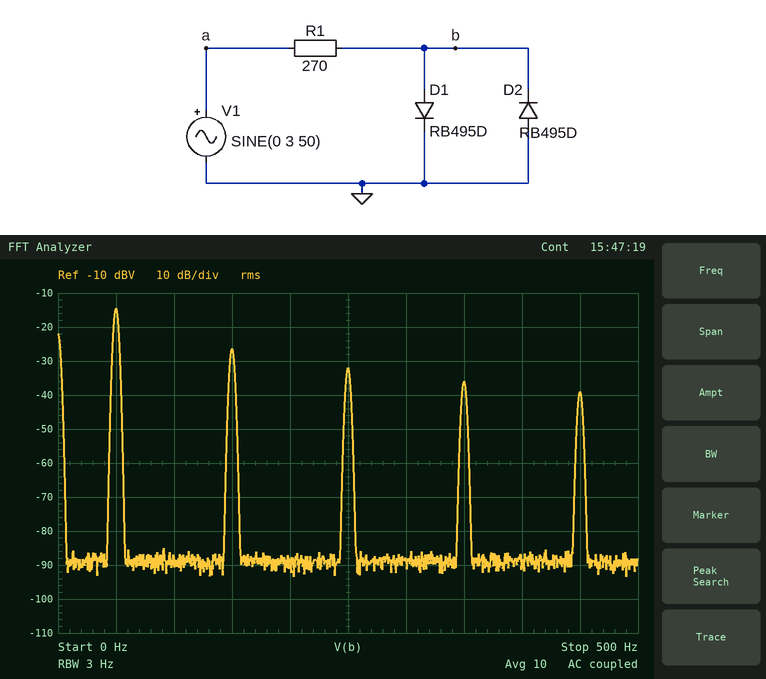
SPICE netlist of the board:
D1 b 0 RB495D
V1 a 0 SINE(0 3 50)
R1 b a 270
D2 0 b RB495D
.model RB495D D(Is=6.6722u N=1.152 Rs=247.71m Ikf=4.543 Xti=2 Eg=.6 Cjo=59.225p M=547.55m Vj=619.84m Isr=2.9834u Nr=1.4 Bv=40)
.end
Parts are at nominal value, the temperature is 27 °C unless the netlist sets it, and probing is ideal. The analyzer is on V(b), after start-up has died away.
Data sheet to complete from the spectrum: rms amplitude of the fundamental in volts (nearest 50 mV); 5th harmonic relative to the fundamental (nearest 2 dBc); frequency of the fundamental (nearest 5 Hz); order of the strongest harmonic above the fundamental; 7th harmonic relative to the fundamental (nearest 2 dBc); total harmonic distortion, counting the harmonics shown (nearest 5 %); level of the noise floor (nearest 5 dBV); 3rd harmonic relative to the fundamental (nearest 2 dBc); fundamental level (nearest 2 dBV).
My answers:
200 mV
-18 dBc
50 Hz
3
-22 dBc
30 %
-90 dBV
-12 dBc
-14 dBV
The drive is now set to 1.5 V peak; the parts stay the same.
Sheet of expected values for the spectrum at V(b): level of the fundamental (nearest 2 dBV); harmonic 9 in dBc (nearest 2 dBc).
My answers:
-16 dBV
-26 dBc
